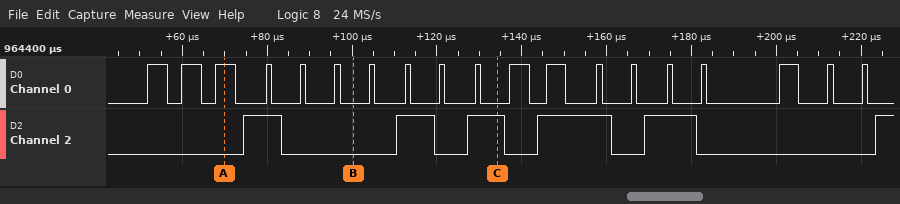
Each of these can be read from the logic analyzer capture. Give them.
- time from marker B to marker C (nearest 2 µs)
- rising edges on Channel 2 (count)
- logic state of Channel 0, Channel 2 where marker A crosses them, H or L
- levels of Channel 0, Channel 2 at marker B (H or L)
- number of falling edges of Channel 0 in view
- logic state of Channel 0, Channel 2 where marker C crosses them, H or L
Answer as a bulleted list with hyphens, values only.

- 34 µs
- 6
- Channel 0=H, Channel 2=L
- Channel 0=L, Channel 2=L
- 19
- Channel 0=L, Channel 2=H
